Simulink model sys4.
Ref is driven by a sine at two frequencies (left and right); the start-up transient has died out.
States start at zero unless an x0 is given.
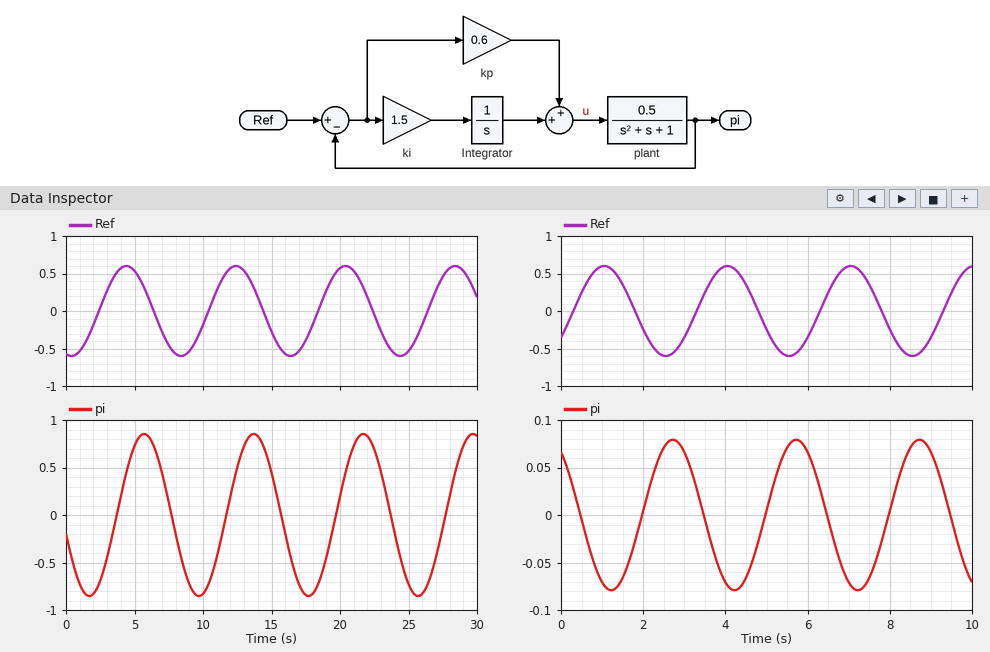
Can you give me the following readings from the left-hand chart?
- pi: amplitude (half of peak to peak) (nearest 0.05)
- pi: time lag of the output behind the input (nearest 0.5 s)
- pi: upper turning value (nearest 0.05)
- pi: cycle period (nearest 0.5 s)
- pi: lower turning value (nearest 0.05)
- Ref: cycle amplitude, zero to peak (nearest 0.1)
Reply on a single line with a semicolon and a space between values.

0.85; 1.5 s; 0.85; 8.0 s; -0.85; 0.6
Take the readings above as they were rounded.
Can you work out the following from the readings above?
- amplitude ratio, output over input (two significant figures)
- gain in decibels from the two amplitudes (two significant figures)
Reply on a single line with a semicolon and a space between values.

1.4; 3.0 dB
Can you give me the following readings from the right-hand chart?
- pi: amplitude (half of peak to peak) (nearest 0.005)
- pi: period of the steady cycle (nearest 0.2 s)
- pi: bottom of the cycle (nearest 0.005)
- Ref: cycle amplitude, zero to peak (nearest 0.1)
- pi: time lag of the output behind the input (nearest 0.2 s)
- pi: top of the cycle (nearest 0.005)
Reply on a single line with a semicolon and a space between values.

0.080; 3.0 s; -0.080; 0.6; 1.6 s; 0.080
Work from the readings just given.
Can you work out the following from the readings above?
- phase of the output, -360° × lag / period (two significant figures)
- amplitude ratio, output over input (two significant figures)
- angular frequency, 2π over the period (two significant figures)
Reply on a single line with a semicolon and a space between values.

-190°; 0.13; 2.1 rad/s
